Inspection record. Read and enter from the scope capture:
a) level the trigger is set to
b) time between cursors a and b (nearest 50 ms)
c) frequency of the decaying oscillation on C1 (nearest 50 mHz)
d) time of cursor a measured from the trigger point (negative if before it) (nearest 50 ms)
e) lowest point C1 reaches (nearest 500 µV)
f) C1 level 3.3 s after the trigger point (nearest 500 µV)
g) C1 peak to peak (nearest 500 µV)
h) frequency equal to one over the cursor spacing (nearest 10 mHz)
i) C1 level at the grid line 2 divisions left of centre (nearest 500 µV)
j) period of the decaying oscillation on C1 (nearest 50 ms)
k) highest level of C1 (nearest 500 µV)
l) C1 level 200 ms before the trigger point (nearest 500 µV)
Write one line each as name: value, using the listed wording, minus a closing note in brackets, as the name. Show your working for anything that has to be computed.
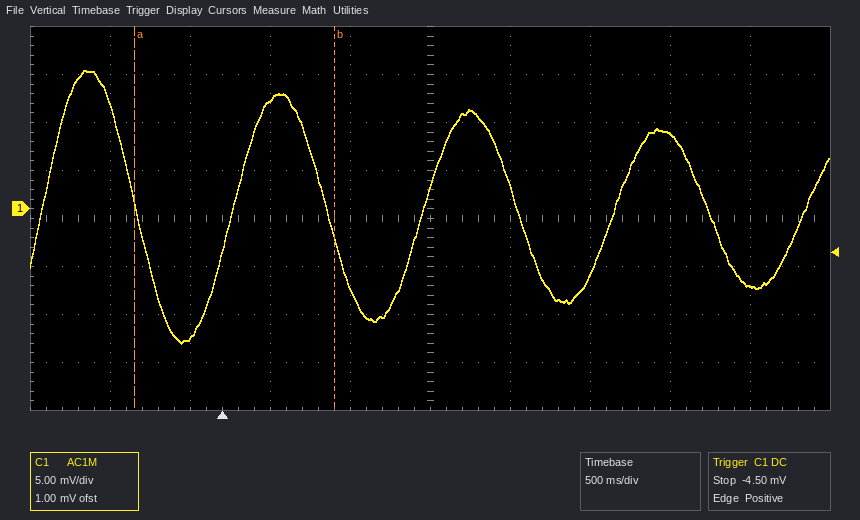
level the trigger is set to: -4.50 mV
time between cursors a and b: 1.25 s
frequency of the decaying oscillation on C1: 1 / 1.20 s ≈ 833 mHz, so 850 mHz to the nearest 50 mHz
time of cursor a measured from the trigger point (negative if before it): -550 ms
lowest point C1 reaches: -14.0 mV
C1 level 3.3 s after the trigger point: -8.0 mV
C1 peak to peak: 14.5 mV − (-14.0 mV) = 28.5 mV
frequency equal to one over the cursor spacing: 1 / 1.25 s ≈ 800 mHz
C1 level at the grid line 2 divisions left of centre: 11.5 mV
period of the decaying oscillation on C1: 1.20 s
highest level of C1: 14.5 mV
C1 level 200 ms before the trigger point: -13.5 mV
